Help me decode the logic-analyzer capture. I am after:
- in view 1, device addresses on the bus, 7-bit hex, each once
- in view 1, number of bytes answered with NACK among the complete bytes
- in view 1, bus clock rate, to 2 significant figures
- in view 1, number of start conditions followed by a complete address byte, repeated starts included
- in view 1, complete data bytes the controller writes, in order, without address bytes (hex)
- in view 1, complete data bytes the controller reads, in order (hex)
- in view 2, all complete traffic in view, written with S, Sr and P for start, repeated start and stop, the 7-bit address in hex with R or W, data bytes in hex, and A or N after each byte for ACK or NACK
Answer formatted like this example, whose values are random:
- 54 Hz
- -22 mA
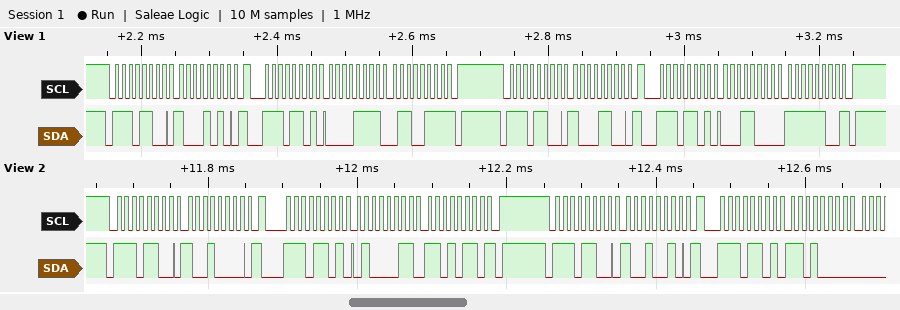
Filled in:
- 0x76
- 2
- 100 kHz
- 4
- 8A 8C
- 0F 67 18 FC
- S 76W A 90 A Sr 76R A 43 A D6 N P S 76W A 92 A Sr 76R A D0 A
